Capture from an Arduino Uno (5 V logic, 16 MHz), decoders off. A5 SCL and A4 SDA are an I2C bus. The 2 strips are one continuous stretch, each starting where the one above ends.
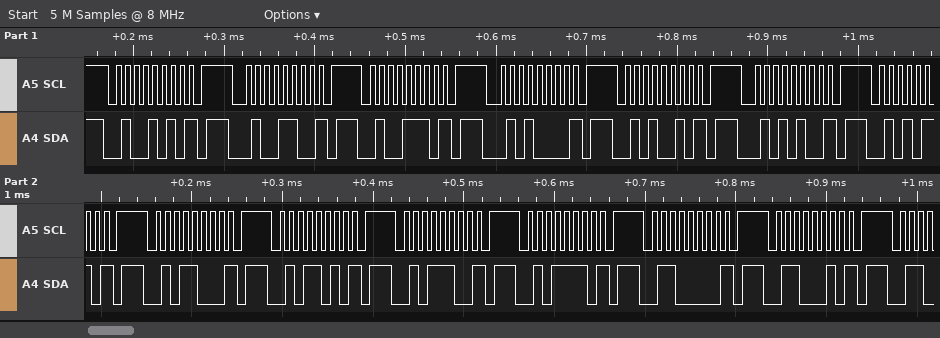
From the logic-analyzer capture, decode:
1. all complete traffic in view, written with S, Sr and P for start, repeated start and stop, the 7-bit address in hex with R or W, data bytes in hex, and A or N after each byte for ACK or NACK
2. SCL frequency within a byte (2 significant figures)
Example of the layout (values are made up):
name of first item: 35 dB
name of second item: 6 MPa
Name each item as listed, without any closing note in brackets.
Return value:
all complete traffic in view, written with S, Sr and P for start, repeated start and stop, the 7-bit address in hex with R or W, data bytes in hex, and A or N after each byte for ACK or NACK: S 25W N P S 26W N P S 27W N P S 28W N P S 29W N P S 2AW N P S 2BW N P S 2CW N P S 2DW N P S 2EW N P S 2FW N P S 30W N P S 31W N P
SCL frequency within a byte: 100 kHz
